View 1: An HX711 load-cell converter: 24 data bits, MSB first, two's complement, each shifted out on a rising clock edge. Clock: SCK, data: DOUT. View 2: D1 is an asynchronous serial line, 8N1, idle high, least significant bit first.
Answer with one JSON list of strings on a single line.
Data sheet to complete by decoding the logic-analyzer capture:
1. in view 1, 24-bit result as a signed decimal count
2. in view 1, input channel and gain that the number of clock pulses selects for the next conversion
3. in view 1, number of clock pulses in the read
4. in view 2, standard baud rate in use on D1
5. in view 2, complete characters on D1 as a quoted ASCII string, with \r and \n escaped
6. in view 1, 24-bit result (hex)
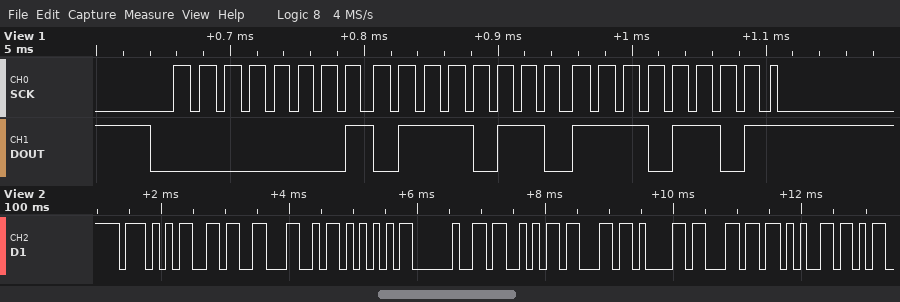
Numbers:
["95981", "channel A, gain 128", "25", "9600 baud", "\"W6LU Scale\"", "0x0176ED"]
